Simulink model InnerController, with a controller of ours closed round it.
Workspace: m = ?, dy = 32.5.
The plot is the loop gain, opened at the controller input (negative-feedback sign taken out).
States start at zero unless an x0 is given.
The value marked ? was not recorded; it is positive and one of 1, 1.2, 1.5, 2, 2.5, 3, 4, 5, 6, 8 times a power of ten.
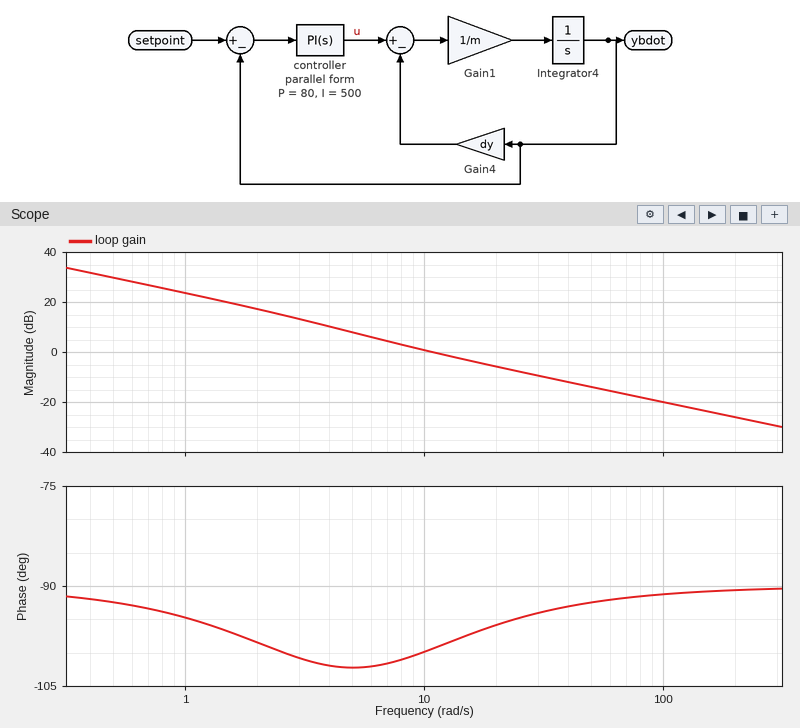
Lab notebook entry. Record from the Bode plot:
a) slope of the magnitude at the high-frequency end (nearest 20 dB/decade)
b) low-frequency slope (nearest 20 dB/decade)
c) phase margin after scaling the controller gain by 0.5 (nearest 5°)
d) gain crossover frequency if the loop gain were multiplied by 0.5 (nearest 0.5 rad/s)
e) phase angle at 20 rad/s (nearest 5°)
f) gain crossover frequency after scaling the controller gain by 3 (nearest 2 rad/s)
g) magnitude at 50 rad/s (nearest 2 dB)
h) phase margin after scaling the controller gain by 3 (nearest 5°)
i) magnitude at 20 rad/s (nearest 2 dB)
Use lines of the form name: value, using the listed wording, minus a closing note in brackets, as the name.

slope of the magnitude at the high-frequency end: -20 dB/decade
low-frequency slope: -20 dB/decade
phase margin after scaling the controller gain by 0.5: 80°
gain crossover frequency if the loop gain were multiplied by 0.5: 6.0 rad/s
phase angle at 20 rad/s: -95°
gain crossover frequency after scaling the controller gain by 3: 30 rad/s
magnitude at 50 rad/s: -14 dB
phase margin after scaling the controller gain by 3: 85°
magnitude at 20 rad/s: -6 dB
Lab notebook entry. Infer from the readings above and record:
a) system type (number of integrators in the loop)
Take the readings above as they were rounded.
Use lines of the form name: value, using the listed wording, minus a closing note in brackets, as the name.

system type: 1
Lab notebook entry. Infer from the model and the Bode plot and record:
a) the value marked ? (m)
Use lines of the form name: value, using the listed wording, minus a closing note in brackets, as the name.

the value marked ?: 8
